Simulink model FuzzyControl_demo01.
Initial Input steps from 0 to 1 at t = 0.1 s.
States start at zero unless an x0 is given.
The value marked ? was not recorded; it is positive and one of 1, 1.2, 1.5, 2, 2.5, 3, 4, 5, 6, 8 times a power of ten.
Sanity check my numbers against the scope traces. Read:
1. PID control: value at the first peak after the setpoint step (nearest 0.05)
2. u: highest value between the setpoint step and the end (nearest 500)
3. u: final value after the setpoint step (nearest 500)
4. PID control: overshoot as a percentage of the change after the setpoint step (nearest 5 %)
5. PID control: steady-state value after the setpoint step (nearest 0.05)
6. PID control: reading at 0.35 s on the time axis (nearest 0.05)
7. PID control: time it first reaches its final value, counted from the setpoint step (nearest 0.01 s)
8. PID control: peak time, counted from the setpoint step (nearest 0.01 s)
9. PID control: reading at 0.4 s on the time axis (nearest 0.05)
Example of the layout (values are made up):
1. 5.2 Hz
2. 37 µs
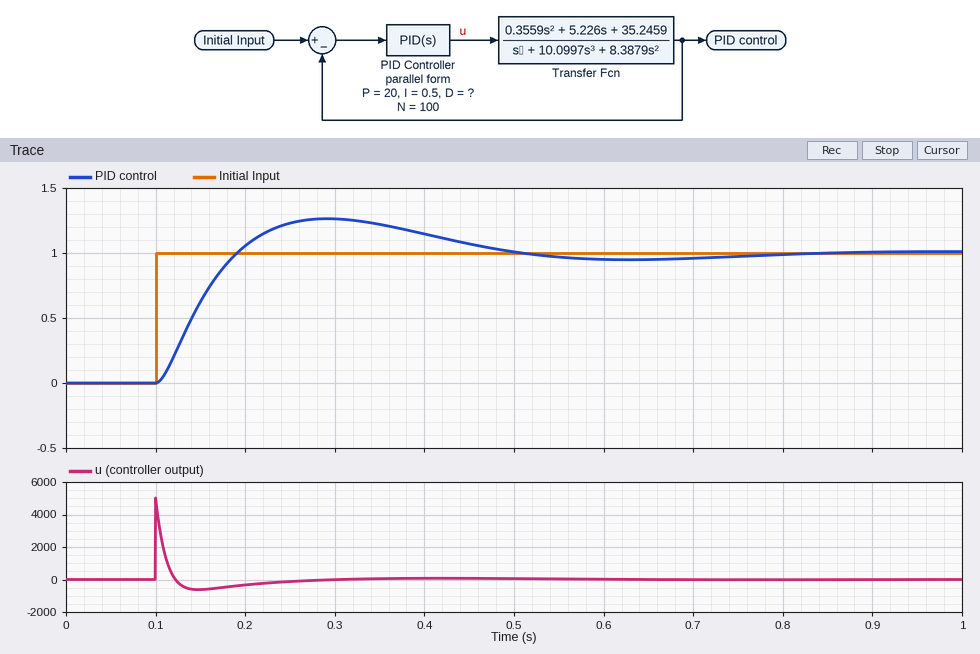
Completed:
1. 1.25
2. 5000
3. 0
4. 25 %
5. 1.00
6. 1.20
7. 0.09 s
8. 0.19 s
9. 1.15
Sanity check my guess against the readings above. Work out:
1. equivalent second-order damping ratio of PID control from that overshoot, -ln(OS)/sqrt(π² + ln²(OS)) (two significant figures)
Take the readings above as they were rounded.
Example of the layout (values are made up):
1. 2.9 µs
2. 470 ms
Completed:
1. 0.40
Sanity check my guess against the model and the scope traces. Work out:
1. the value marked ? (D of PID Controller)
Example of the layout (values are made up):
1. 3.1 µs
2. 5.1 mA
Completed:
1. 50
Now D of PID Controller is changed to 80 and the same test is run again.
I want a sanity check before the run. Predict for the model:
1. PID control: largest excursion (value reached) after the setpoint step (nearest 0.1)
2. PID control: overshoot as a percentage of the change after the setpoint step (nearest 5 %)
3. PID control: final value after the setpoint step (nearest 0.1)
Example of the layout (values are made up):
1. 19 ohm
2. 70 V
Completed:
1. 1.2
2. 20 %
3. 1.0
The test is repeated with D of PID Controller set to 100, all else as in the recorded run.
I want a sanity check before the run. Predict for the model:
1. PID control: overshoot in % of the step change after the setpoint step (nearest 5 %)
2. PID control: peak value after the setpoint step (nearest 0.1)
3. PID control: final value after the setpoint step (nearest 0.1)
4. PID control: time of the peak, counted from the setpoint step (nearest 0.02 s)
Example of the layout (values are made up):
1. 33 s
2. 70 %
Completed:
1. 15 %
2. 1.2
3. 1.0
4. 0.10 s
